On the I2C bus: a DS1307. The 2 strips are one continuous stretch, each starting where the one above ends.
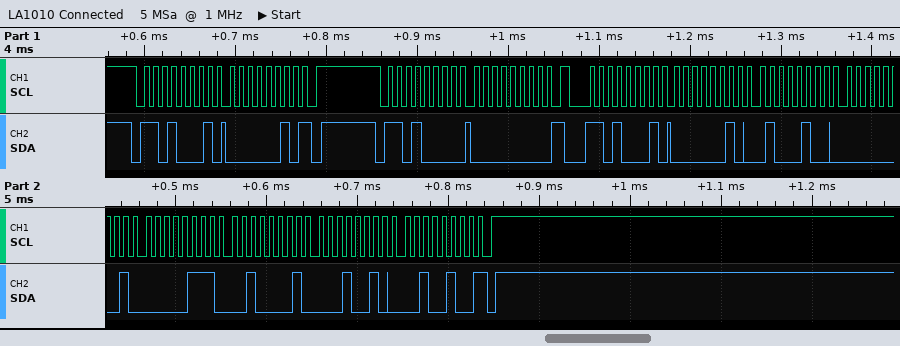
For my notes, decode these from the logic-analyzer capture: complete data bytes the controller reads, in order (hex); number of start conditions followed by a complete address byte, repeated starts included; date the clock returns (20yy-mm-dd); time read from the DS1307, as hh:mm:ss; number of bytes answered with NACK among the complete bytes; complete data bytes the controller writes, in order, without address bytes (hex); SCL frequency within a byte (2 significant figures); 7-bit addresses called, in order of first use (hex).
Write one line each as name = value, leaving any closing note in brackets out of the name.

complete data bytes the controller reads, in order = 02 02 44 01 07 21 12 24
number of start conditions followed by a complete address byte, repeated starts included = 3
date the clock returns = 2024-12-21
time read from the DS1307, as hh:mm:ss = 01:44:02
number of bytes answered with NACK among the complete bytes = 2
complete data bytes the controller writes, in order, without address bytes = 00
SCL frequency within a byte = 100 kHz
7-bit addresses called, in order of first use = 0x68
